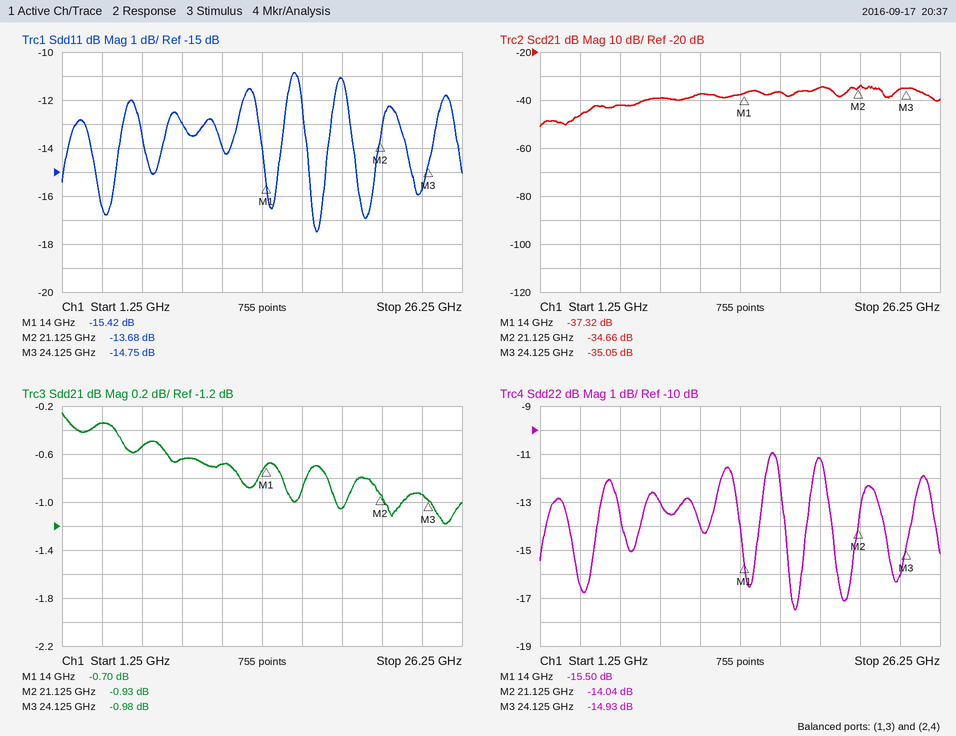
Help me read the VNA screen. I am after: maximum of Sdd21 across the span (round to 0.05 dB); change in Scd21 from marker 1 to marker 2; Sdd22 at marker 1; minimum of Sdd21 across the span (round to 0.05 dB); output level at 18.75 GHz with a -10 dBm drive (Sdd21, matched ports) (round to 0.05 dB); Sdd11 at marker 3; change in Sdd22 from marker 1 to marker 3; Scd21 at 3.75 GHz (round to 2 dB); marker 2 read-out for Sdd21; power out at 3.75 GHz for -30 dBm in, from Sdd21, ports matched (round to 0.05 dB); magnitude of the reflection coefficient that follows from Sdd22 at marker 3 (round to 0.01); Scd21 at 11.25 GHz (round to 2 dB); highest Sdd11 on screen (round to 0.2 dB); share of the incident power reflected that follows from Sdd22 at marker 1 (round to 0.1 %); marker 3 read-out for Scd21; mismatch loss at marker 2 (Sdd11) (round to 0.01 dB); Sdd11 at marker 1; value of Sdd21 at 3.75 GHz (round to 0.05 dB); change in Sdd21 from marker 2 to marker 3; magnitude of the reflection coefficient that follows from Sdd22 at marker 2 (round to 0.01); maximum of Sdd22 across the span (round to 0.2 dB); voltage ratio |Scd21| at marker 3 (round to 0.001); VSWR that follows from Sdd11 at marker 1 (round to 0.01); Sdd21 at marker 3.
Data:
-0.25 dB
2.66 dB
-15.50 dB
-1.20 dB
-11.05 dBm
-14.75 dB
0.57 dB
-46 dB
-0.93 dB
-30.35 dBm
0.18
-38 dB
-10.8 dB
2.8 %
-35.05 dB
0.19 dB
-15.42 dB
-0.35 dB
-0.05 dB
0.20
-11.0 dB
0.018
1.41
-0.98 dB
